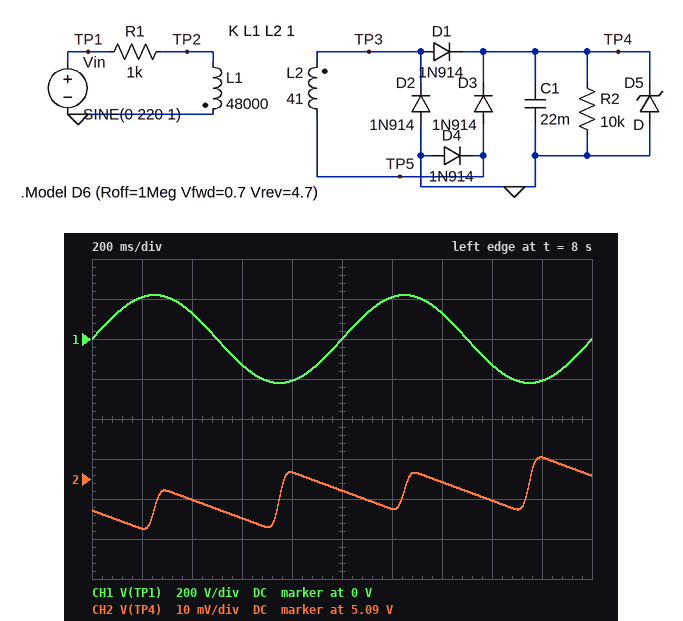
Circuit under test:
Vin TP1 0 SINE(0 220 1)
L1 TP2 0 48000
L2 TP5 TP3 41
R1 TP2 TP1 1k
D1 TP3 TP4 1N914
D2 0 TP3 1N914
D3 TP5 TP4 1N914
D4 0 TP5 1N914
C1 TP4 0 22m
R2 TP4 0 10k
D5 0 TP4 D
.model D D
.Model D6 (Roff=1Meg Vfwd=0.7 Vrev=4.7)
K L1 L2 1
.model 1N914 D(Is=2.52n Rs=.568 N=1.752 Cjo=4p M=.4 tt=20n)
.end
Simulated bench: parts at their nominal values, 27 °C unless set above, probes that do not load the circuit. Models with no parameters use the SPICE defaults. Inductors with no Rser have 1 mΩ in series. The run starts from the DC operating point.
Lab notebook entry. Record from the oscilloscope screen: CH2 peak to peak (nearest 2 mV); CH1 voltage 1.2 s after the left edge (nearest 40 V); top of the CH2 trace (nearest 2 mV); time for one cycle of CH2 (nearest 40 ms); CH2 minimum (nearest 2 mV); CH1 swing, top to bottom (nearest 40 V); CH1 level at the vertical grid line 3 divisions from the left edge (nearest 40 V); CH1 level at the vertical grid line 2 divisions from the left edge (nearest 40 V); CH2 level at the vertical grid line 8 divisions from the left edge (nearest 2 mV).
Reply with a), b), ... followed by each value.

a) 18 mV
b) 200 V
c) 5.096 V
d) 480 ms
e) 5.078 V
f) 440 V
g) -120 V
h) 120 V
i) 5.084 V
